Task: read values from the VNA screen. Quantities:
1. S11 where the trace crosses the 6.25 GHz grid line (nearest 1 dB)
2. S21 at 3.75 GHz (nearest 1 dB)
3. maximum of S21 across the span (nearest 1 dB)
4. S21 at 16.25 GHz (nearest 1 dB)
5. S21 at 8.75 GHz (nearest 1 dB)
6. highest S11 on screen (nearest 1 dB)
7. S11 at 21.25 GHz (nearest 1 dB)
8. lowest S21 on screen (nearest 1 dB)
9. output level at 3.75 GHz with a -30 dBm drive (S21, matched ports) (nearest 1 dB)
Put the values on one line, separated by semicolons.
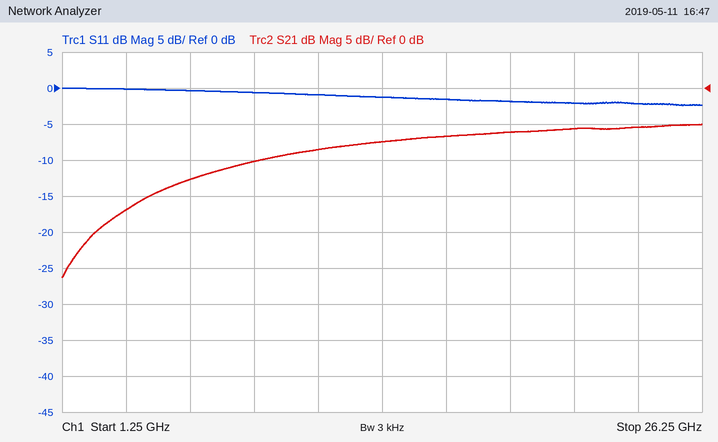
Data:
0 dB; -17 dB; -5 dB; -7 dB; -10 dB; 0 dB; -2 dB; -26 dB; -47 dBm
